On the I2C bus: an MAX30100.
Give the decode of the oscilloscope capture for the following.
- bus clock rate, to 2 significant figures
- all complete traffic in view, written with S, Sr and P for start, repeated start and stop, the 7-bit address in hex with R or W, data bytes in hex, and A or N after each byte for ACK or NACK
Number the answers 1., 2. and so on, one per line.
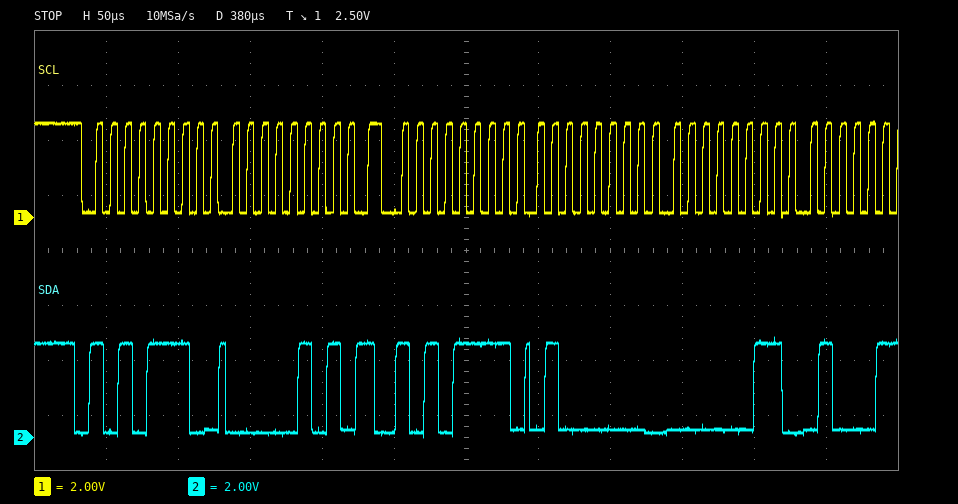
1. 100 kHz
2. S 57W A 05 A Sr 57R A 40 A 03 A
